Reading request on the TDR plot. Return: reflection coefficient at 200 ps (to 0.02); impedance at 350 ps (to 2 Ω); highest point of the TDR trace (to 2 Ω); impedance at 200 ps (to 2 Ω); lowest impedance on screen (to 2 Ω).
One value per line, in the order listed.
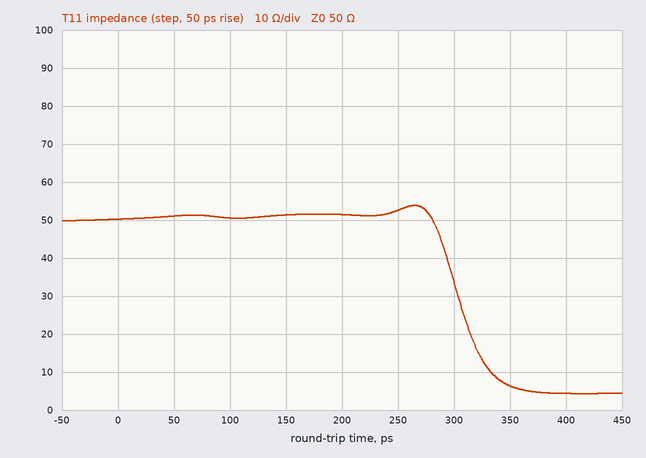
+0.02
6 Ω
54 Ω
52 Ω
4 Ω
